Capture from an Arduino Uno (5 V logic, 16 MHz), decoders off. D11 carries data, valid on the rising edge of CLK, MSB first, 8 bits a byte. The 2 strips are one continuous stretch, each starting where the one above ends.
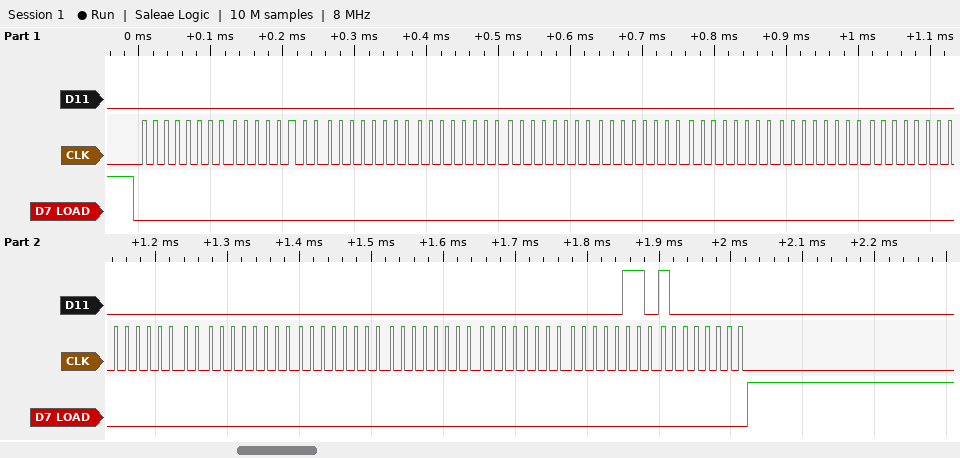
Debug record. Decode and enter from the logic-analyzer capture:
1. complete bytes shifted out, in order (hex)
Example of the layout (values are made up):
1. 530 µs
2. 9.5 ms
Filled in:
1. 0x00 0x00 0x00 0x00 0x00 0x00 0x00 0x00 0x00 0x00 0x00 0x00 0x00 0x00 0x06 0x80
